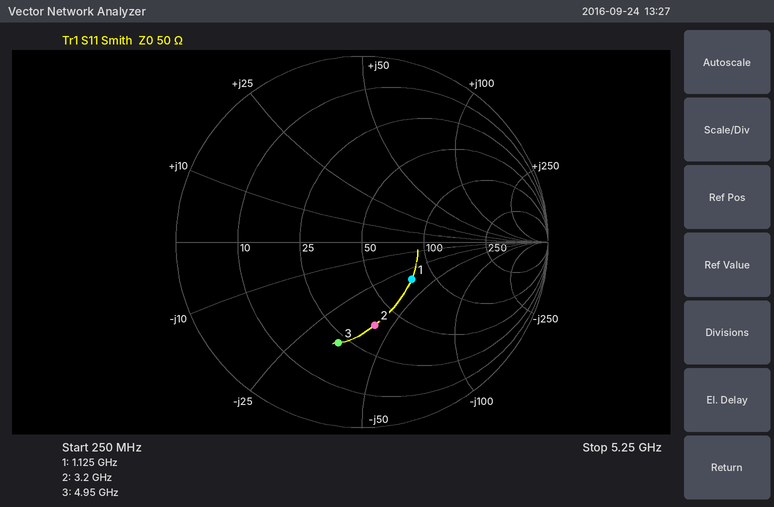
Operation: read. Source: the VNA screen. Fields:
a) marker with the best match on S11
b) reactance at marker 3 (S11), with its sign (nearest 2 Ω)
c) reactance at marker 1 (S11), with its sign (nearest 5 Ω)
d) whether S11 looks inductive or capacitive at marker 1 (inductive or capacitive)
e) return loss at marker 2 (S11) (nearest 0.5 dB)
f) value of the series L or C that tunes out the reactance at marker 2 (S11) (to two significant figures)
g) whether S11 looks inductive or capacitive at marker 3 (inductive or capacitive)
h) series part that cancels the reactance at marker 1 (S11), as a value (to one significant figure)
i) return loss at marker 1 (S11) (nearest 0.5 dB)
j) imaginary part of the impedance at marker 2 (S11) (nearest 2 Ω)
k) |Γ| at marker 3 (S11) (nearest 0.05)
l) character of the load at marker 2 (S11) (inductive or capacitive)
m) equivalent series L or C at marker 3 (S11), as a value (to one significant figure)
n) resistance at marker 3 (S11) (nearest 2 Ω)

marker 1
-34 Ω
-35 Ω
capacitive
7.0 dB
2.1 nH
capacitive
5 nH
9.5 dB
-42 Ω
0.55
capacitive
900 fF
22 Ω
